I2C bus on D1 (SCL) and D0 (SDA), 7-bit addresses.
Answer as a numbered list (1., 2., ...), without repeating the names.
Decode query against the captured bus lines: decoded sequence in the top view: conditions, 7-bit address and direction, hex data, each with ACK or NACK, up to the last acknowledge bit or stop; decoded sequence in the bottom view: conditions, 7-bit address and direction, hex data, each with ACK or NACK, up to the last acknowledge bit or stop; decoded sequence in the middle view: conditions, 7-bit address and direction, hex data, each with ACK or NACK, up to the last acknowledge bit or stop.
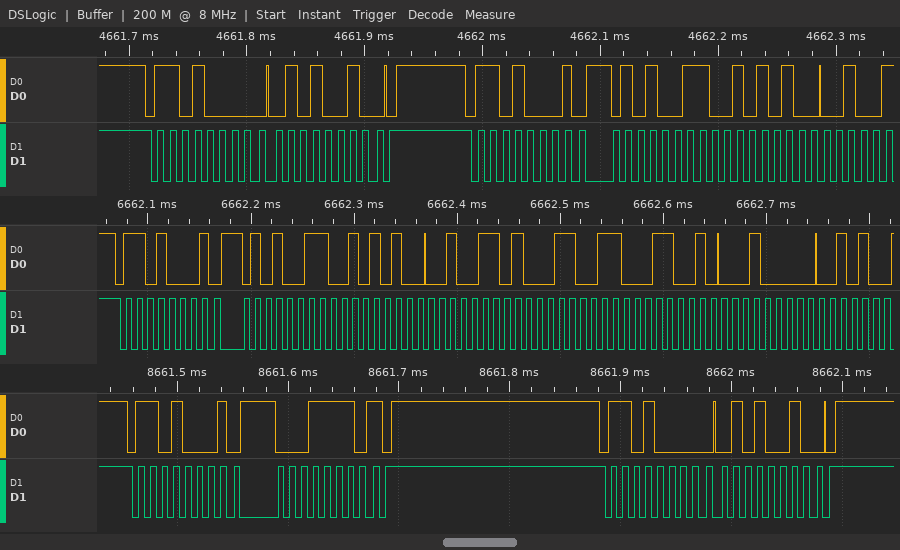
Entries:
1. start, address 68 write ACK, 52 ACK, stop, start, address 68 read ACK, 53 ACK, 54 ACK
2. start, address 68 read ACK, 1E NACK, stop, start, address 68 write ACK, 52 ACK, stop
3. start, address 68 read ACK, 53 ACK, 54 ACK, 4D ACK, 33 ACK, 32 ACK, 20 ACK
